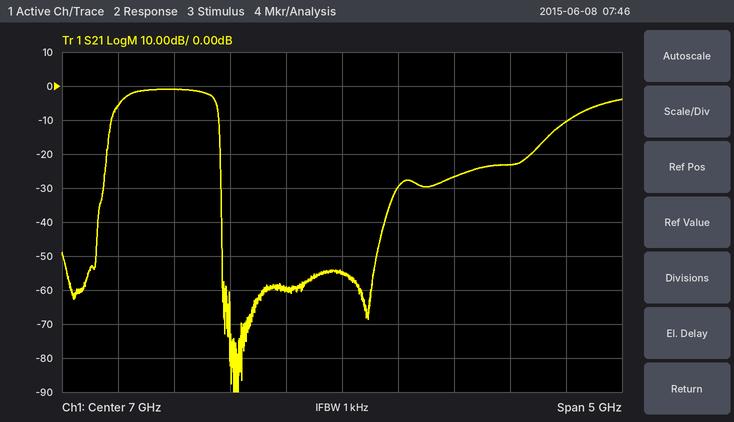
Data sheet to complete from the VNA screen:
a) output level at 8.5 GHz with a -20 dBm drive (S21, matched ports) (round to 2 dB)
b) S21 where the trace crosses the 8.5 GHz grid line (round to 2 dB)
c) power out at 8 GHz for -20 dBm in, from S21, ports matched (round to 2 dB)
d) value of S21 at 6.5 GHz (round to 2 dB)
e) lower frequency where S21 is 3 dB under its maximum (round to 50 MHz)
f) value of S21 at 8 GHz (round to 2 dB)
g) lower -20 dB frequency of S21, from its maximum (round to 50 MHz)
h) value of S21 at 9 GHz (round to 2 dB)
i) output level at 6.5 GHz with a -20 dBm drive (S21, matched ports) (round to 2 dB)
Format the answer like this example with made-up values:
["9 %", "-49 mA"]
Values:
["-44 dBm", "-24 dB", "-46 dBm", "-60 dB", "5.05 GHz", "-26 dB", "4.90 GHz", "-10 dB", "-80 dBm"]
